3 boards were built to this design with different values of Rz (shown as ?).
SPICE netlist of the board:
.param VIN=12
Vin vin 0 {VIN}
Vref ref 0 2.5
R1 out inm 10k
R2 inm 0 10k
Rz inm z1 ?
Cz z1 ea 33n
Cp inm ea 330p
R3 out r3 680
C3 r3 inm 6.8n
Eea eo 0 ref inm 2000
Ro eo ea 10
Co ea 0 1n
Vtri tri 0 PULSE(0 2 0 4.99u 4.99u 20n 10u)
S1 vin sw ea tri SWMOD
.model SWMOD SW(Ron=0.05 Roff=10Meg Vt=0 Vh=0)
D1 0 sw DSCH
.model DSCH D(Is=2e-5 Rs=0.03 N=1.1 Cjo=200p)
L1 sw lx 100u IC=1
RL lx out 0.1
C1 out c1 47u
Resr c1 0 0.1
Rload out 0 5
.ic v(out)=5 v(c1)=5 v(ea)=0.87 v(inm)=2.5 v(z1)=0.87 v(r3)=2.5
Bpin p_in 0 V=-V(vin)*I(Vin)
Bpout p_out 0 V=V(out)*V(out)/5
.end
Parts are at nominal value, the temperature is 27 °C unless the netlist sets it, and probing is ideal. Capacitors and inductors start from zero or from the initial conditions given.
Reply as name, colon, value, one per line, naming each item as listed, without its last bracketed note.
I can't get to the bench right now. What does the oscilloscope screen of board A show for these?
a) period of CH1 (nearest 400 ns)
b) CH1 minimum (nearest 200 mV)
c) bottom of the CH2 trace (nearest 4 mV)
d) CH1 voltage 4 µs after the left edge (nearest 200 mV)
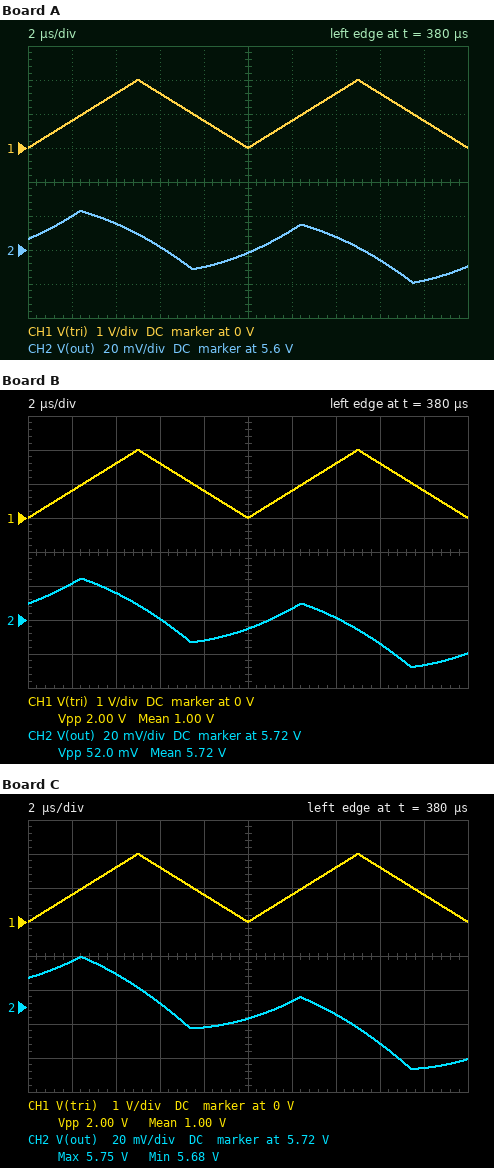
period of CH1: 10.0 µs
CH1 minimum: 0 V
bottom of the CH2 trace: 5.580 V
CH1 voltage 4 µs after the left edge: 1.6 V
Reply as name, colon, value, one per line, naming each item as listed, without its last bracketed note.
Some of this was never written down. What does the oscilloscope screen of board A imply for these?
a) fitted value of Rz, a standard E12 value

fitted value of Rz, a standard E12 value: 18 kΩ
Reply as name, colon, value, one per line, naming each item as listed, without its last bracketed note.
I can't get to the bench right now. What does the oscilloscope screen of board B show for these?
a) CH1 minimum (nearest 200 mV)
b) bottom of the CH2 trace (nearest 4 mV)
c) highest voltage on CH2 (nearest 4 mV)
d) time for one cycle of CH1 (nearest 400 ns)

CH1 minimum: 0 V
bottom of the CH2 trace: 5.692 V
highest voltage on CH2: 5.744 V
time for one cycle of CH1: 10.0 µs
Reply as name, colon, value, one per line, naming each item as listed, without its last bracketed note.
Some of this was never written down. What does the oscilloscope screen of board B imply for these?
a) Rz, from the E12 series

Rz, from the E12 series: 12 kΩ
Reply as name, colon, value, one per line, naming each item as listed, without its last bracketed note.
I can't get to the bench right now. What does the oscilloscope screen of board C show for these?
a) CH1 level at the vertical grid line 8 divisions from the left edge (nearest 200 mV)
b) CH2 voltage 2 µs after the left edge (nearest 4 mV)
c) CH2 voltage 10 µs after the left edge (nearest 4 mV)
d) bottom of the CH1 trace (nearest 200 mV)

CH1 level at the vertical grid line 8 divisions from the left edge: 1.6 V
CH2 voltage 2 µs after the left edge: 5.748 V
CH2 voltage 10 µs after the left edge: 5.712 V
bottom of the CH1 trace: 0 V
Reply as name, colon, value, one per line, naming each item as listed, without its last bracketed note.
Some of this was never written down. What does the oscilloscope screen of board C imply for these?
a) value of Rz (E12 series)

value of Rz: 6.8 kΩ
